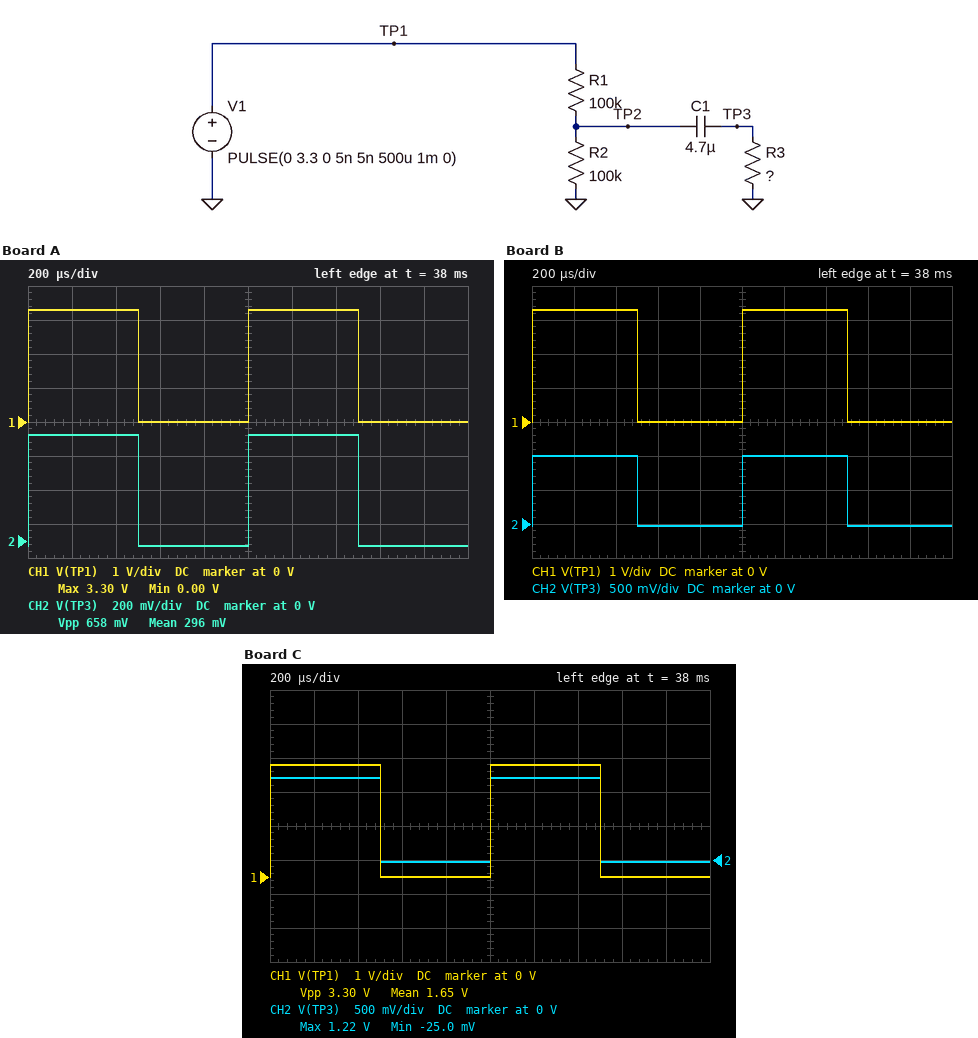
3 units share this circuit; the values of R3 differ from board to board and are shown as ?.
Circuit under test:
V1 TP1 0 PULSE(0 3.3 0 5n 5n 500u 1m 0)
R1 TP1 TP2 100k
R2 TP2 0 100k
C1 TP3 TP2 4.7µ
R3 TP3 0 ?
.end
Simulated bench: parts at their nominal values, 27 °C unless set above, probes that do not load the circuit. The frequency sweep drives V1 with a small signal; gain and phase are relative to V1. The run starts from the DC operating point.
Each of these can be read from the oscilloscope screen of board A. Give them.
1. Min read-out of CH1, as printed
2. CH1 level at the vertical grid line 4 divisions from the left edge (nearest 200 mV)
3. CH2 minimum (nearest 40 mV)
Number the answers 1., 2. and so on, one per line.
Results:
1. 0.00 V
2. 0 V
3. -40 mV
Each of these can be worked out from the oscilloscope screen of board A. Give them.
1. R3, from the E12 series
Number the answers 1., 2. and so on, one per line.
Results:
1. 33 kΩ
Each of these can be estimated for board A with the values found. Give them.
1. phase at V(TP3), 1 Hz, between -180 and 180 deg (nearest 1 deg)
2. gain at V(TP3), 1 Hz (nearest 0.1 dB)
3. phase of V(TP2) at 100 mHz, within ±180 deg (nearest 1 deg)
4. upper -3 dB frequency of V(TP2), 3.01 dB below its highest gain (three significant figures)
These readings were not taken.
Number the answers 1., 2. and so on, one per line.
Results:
1. 22 deg
2. -14.7 dB
3. -8 deg
4. 493 mHz
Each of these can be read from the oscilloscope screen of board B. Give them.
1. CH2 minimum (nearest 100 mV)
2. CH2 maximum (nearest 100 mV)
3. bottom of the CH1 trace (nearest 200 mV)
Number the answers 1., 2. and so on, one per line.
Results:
1. 0 V
2. 1.0 V
3. 0 V
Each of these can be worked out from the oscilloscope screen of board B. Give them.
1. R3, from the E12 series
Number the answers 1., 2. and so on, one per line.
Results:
1. 82 kΩ
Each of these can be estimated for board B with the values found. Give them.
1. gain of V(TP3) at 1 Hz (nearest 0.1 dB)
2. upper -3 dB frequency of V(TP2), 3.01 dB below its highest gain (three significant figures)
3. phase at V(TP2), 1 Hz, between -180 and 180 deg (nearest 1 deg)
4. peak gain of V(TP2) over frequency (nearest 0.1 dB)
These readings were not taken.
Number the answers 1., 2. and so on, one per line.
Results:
1. -10.4 dB
2. 537 mHz
3. -8 deg
4. -6.0 dB
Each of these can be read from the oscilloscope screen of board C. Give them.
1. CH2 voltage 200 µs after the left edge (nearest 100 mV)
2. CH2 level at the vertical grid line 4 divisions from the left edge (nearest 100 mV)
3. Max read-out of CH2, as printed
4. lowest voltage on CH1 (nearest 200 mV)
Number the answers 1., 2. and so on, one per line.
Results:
1. 1.2 V
2. 0 V
3. 1.22 V
4. 0 V
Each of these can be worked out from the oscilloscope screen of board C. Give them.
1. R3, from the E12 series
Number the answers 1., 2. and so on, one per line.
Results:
1. 150 kΩ
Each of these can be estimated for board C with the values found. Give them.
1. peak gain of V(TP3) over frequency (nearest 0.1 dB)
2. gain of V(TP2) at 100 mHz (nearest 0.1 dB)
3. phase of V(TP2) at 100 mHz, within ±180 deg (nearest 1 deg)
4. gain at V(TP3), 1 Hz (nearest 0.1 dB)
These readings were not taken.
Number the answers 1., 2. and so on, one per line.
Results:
1. -8.5 dB
2. -6.5 dB
3. -7 deg
4. -8.6 dB
